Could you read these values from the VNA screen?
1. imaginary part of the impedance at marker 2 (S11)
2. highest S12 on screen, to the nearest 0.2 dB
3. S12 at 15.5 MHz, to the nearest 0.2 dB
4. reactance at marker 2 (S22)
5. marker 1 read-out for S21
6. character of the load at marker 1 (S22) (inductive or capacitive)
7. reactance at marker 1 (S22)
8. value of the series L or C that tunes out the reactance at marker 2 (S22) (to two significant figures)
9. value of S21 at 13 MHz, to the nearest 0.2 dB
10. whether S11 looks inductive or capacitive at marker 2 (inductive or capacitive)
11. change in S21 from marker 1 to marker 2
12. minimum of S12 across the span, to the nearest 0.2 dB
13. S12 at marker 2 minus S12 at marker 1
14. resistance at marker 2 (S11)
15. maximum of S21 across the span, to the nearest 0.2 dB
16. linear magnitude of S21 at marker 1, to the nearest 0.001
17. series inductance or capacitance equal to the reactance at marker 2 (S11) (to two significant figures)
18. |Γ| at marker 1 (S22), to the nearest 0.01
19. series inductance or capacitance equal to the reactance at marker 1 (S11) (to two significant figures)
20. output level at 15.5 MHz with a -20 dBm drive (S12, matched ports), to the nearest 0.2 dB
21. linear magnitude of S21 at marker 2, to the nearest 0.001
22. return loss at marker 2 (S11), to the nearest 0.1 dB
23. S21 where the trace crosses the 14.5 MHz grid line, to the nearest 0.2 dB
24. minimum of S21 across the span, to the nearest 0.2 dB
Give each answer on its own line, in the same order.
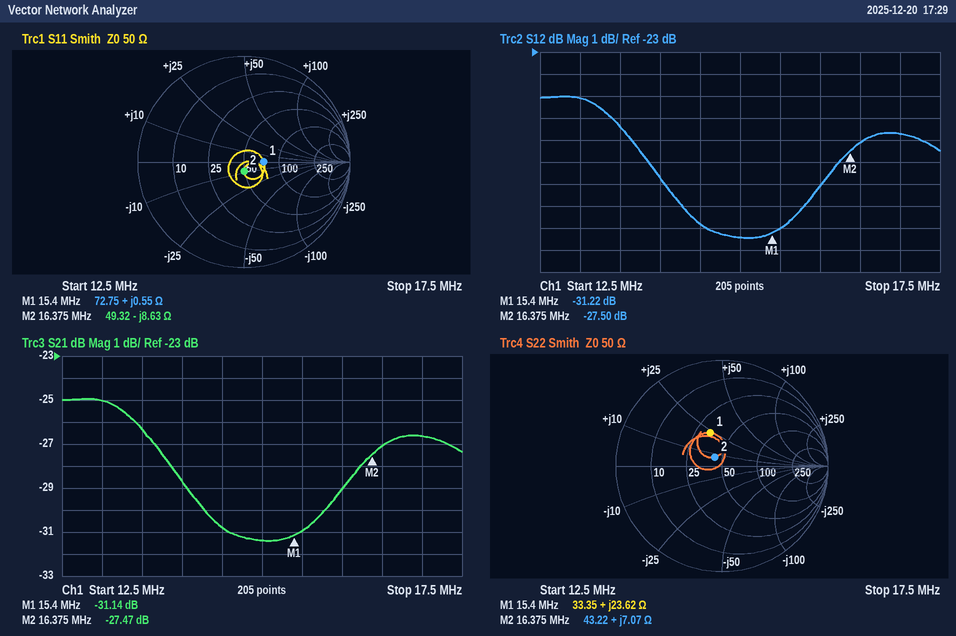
-8.63 Ω
-25.0 dB
-31.0 dB
+7.07 Ω
-31.14 dB
inductive
+23.62 Ω
1.4 nF
-25.0 dB
capacitive
3.67 dB
-31.4 dB
3.72 dB
49.32 Ω
-25.0 dB
0.028
1.1 nF
0.33
5.7 nH
-51.0 dBm
0.042
21.2 dB
-30.8 dB
-31.4 dB
